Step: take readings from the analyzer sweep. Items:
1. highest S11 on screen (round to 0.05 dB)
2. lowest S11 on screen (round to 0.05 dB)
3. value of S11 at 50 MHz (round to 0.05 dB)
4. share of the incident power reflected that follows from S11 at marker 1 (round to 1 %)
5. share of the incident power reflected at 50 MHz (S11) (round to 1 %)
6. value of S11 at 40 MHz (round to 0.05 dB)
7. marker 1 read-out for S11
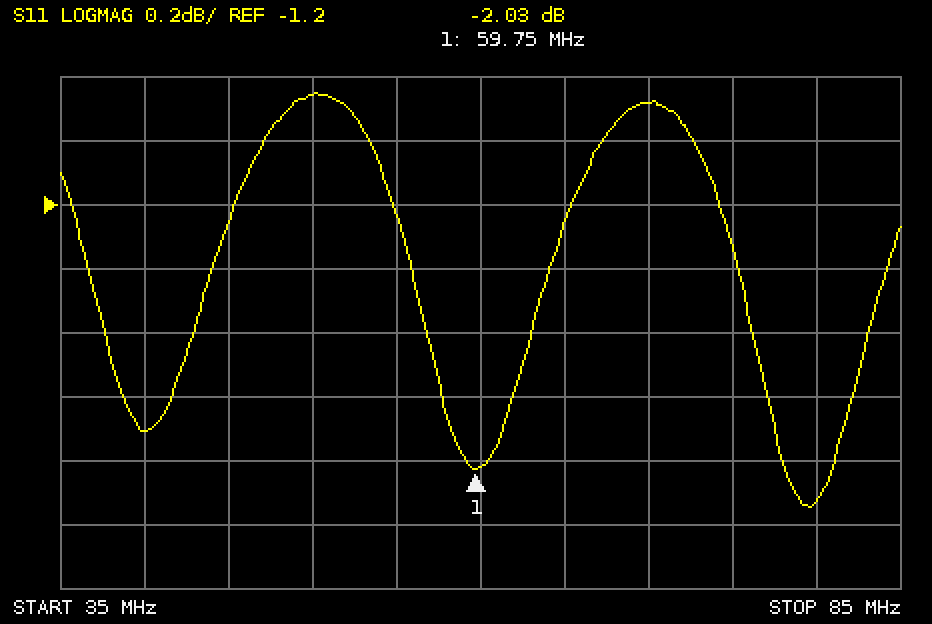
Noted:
-0.85 dB
-2.15 dB
-0.85 dB
63 %
82 %
-1.90 dB
-2.03 dB
